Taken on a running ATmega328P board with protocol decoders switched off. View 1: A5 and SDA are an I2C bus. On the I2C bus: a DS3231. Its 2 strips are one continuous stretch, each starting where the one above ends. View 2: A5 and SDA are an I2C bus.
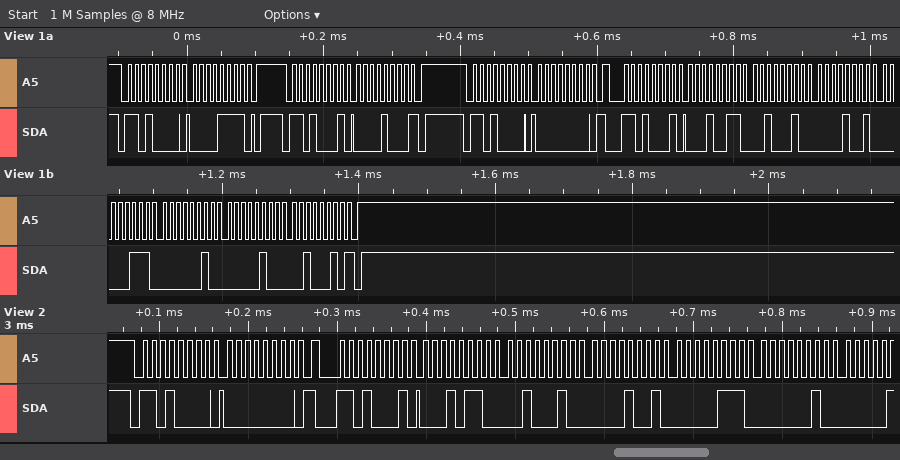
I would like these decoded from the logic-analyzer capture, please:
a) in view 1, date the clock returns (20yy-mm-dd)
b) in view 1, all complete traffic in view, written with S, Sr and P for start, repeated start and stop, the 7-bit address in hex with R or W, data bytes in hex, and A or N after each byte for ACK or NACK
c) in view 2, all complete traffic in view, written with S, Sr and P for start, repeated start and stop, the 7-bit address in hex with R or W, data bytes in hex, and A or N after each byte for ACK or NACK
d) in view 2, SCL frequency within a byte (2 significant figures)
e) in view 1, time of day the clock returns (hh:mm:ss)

2022-04-02
S 68W A 0F A P S 68R A 08 N P S 68W A 00 A Sr 68R A 13 A 22 A 09 A 07 A 02 A 04 A 22 N P
S 68W A 00 A Sr 68R A 16 A 22 A 09 A 07 A 02 A
100 kHz
09:22:13
